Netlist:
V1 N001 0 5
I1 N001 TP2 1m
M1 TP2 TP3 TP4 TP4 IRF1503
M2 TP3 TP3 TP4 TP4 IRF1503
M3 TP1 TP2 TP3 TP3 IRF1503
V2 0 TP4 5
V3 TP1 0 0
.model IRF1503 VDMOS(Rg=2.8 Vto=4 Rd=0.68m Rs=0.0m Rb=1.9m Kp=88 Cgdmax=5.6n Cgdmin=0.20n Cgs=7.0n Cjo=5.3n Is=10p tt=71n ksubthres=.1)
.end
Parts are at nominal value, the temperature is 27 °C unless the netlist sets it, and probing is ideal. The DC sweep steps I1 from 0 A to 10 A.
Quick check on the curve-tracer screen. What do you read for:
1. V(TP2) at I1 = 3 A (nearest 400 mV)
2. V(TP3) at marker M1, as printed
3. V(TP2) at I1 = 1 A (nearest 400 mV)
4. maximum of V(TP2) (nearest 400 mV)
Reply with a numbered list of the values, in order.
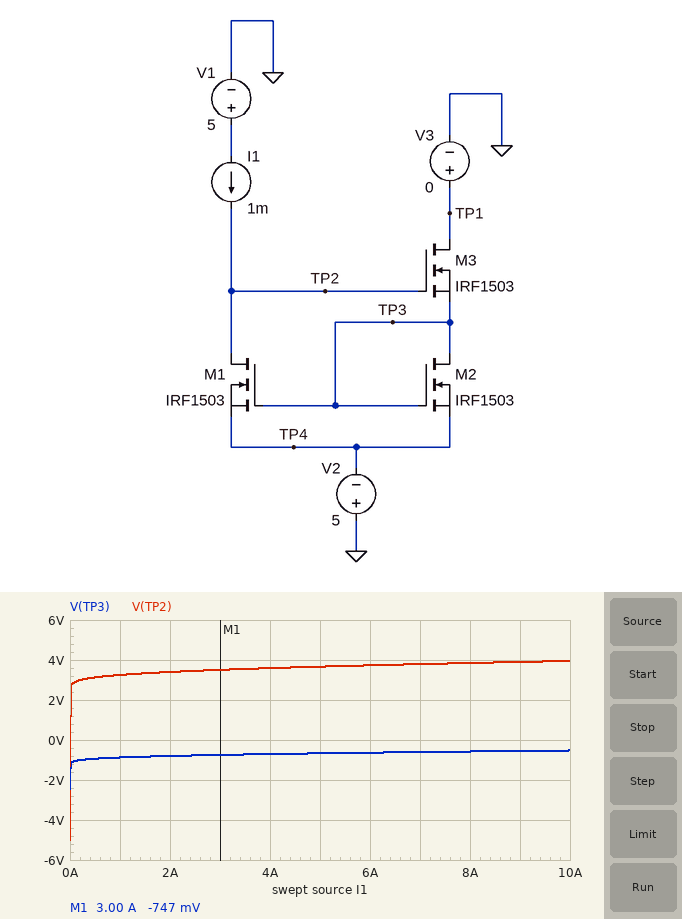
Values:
1. 3.6 V
2. -747 mV
3. 3.2 V
4. 4.0 V
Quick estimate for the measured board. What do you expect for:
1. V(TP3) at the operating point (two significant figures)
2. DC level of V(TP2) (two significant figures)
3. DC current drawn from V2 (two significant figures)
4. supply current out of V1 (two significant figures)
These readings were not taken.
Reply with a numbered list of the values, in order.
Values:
1. -1.3 V
2. 2.4 V
3. 2.0 mA
4. 1.0 mA
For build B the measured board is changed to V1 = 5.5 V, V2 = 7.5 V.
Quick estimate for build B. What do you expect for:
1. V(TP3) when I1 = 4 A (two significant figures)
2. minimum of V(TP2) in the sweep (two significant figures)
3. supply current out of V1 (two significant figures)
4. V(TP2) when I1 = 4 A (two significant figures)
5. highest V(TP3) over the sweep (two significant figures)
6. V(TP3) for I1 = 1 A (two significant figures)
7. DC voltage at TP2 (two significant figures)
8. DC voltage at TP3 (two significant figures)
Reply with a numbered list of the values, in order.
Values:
1. -3.2 V
2. -7.5 V
3. 1.0 mA
4. 1.1 V
5. -3.0 V
6. -3.4 V
7. -100 mV
8. -3.8 V
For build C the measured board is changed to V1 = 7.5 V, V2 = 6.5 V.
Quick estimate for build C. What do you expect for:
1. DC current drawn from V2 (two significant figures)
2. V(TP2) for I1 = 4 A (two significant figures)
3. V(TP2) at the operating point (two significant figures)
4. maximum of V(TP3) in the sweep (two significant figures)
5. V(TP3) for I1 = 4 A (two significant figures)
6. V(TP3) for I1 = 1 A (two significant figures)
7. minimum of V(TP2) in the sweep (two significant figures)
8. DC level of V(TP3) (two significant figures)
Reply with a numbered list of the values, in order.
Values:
1. 2.0 mA
2. 2.1 V
3. 900 mV
4. -2.0 V
5. -2.2 V
6. -2.4 V
7. -6.5 V
8. -2.8 V
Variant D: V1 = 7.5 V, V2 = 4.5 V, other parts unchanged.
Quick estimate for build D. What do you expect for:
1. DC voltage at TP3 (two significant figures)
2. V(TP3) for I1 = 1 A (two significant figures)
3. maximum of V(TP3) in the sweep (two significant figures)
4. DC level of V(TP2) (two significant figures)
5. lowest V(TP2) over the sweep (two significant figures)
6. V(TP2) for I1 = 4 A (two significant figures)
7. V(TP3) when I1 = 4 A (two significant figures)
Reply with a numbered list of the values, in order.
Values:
1. -800 mV
2. -370 mV
3. -24 mV
4. 2.9 V
5. -4.5 V
6. 4.1 V
7. -200 mV
